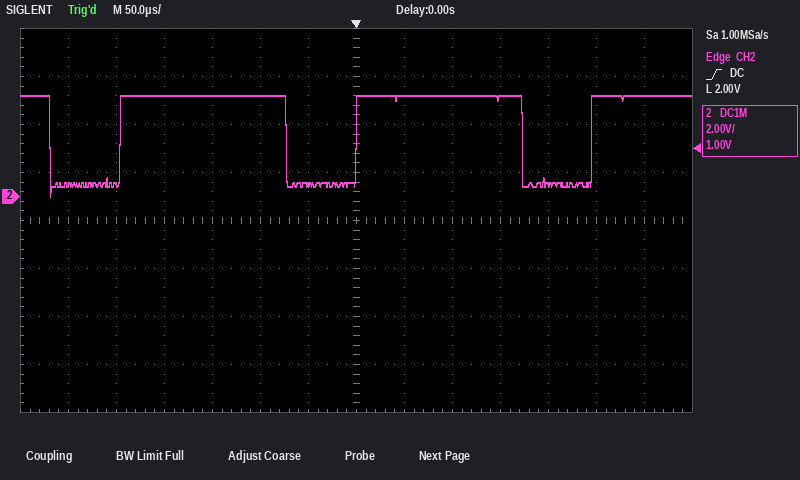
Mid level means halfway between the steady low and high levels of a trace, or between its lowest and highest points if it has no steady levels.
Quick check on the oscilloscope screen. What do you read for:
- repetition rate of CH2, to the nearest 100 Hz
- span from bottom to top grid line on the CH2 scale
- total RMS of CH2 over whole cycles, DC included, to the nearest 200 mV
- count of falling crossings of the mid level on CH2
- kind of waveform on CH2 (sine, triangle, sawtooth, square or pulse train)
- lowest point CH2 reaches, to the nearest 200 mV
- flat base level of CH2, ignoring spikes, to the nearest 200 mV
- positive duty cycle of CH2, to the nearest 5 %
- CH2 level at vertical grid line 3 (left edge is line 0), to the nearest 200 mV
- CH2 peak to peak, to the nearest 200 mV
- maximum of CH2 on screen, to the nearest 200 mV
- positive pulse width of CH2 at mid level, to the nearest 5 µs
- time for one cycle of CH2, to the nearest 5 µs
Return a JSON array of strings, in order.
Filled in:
["4.1 kHz", "16 V", "3.6 V", "3", "pulse train", "0.0 V", "600 mV", "70 %", "4.2 V", "4.2 V", "4.2 V", "175 µs", "245 µs"]
